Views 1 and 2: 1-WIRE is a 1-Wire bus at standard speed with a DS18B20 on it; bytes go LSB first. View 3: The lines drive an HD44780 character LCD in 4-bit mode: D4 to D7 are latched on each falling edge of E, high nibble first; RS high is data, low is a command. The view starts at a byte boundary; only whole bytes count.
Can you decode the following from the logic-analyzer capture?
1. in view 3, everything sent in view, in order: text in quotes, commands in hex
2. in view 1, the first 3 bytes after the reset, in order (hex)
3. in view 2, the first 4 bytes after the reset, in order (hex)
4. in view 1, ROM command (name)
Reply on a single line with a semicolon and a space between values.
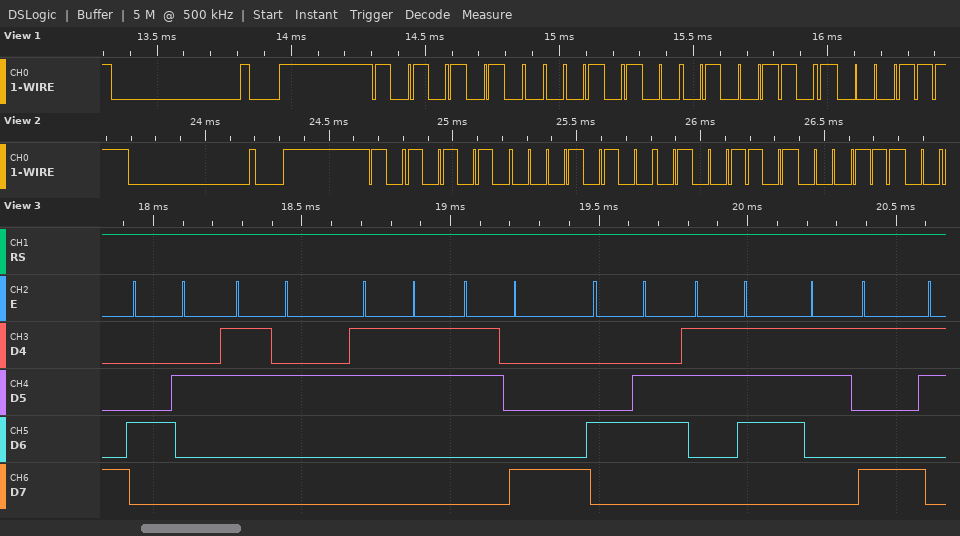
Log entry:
"B238F79"; 55 28 B2; 55 28 B2 38; Match ROM
